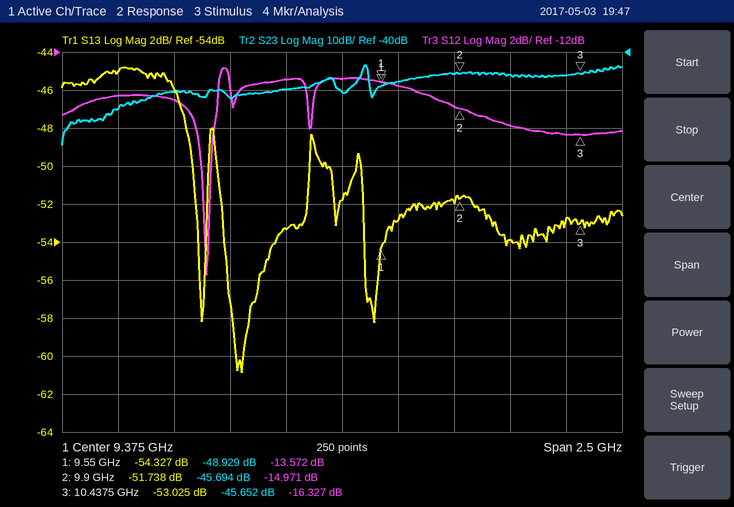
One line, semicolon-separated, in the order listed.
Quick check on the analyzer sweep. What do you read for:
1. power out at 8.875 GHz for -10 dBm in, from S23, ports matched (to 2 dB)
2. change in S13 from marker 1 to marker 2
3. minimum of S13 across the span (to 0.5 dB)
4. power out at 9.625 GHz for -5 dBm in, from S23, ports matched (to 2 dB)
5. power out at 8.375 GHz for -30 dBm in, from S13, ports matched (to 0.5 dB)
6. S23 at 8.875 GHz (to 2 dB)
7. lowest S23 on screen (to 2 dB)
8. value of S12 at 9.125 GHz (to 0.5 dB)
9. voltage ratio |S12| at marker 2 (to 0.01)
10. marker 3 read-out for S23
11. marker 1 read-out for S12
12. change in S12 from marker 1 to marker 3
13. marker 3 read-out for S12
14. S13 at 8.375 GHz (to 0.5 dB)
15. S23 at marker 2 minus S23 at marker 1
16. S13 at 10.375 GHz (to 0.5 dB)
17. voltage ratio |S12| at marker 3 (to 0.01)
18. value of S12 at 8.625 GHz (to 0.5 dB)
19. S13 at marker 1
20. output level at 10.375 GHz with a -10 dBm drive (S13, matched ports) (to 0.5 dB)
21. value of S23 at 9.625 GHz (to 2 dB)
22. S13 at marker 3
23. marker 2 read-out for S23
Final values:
-62 dBm; 2.589 dB; -61.0 dB; -52 dBm; -75.0 dBm; -52 dB; -64 dB; -13.5 dB; 0.18; -45.652 dB; -13.572 dB; -2.755 dB; -16.327 dB; -45.0 dB; 3.235 dB; -53.0 dB; 0.15; -14.5 dB; -54.327 dB; -63.0 dBm; -48 dB; -53.025 dB; -45.694 dB
